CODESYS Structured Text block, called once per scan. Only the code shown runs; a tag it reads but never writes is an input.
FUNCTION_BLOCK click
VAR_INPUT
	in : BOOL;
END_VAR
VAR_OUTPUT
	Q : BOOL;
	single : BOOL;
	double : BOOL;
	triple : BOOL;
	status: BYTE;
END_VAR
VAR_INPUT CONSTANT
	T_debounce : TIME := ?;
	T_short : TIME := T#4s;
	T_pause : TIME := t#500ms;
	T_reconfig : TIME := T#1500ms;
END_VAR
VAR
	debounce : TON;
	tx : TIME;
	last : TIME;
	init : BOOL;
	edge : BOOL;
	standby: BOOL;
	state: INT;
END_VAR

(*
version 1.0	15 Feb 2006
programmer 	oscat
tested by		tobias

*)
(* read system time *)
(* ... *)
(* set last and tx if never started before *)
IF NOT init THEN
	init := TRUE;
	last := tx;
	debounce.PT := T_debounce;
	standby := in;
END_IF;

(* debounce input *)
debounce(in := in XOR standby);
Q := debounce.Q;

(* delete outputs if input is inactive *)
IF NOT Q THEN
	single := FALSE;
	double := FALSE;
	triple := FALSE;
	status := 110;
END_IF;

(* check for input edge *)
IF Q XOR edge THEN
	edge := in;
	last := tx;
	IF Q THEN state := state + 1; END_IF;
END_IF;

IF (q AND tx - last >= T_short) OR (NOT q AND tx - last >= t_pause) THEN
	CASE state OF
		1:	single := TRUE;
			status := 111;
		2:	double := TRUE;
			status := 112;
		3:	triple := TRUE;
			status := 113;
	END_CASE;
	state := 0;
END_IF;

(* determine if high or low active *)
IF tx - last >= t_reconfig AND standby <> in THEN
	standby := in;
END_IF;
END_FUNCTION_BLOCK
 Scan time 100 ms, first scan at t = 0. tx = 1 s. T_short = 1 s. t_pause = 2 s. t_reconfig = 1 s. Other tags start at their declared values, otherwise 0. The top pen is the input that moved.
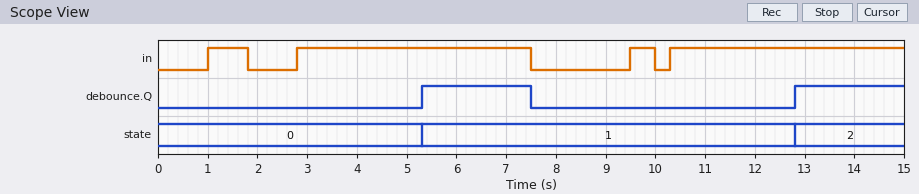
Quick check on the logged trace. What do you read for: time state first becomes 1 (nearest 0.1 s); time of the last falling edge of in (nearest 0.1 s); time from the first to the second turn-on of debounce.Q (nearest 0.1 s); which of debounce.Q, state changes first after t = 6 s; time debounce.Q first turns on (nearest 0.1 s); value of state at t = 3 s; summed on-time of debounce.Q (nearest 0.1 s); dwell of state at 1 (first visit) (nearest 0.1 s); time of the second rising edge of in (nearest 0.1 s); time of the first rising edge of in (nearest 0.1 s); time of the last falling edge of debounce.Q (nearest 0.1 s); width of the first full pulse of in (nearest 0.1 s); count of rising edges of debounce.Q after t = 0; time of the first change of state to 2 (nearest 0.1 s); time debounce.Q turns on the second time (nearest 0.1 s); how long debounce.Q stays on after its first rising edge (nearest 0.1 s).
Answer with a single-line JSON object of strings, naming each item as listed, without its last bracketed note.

{"time state first becomes 1": "5.3 s", "time of the last falling edge of in": "10.0 s", "time from the first to the second turn-on of debounce.Q": "7.5 s", "which of debounce.Q, state changes first after t = 6 s": "debounce.Q", "time debounce.Q first turns on": "5.3 s", "value of state at t = 3 s": "0", "summed on-time of debounce.Q": "4.4 s", "dwell of state at 1 (first visit)": "7.5 s", "time of the second rising edge of in": "2.8 s", "time of the first rising edge of in": "1.0 s", "time of the last falling edge of debounce.Q": "7.5 s", "width of the first full pulse of in": "0.8 s", "count of rising edges of debounce.Q after t = 0": "2", "time of the first change of state to 2": "12.8 s", "time debounce.Q turns on the second time": "12.8 s", "how long debounce.Q stays on after its first rising edge": "2.2 s"}
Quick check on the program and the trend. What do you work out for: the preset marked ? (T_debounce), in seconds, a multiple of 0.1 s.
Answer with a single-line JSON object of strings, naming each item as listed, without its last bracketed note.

{"the preset marked ? (T_debounce), in seconds, a multiple of 0.1 s": "2.5 s"}
